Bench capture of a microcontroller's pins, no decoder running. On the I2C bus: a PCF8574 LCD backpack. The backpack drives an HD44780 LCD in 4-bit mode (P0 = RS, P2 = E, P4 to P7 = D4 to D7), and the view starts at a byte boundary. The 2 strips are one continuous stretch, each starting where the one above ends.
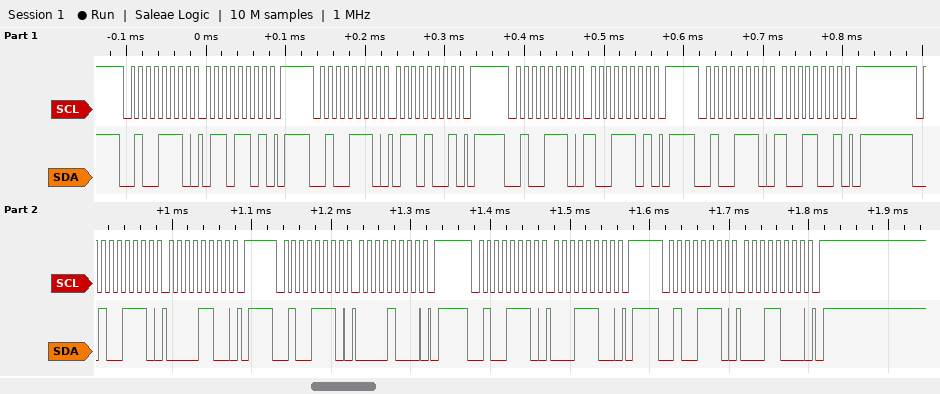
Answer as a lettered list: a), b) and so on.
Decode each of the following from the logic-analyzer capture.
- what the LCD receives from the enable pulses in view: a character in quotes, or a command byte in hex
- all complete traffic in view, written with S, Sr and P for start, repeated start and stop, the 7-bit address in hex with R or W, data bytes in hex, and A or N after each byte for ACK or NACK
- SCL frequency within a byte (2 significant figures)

a) 'i' 0x01
b) S 27W A 6D A P S 27W A 69 A P S 27W A 9D A P S 27W A 99 A P S 27W A 0C A P S 27W A 08 A P S 27W A 1C A P S 27W A 18 A P
c) 100 kHz
